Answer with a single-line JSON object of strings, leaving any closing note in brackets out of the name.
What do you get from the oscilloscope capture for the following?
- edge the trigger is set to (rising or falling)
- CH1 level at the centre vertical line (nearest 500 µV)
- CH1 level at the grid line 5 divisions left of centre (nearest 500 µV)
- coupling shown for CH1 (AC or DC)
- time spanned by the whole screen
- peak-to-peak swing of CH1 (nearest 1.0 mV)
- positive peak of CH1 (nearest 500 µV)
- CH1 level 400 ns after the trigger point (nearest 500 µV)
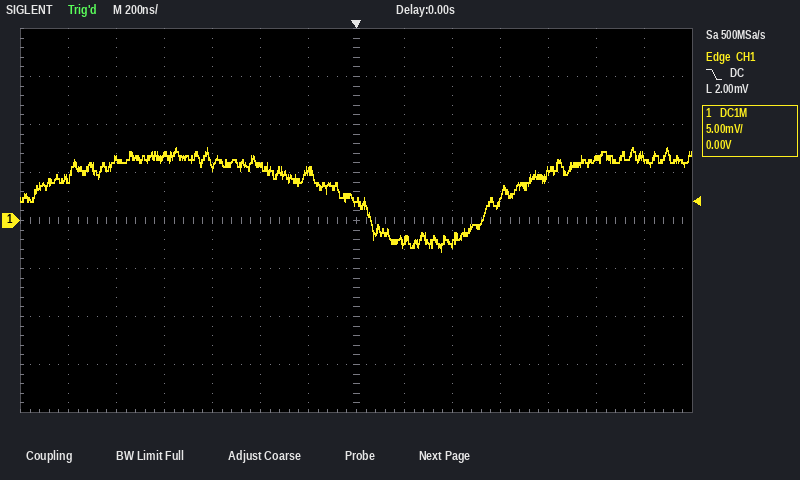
{"edge the trigger is set to": "falling", "CH1 level at the centre vertical line": "2.0 mV", "CH1 level at the grid line 5 divisions left of centre": "6.5 mV", "coupling shown for CH1": "DC", "time spanned by the whole screen": "2.8 µs", "peak-to-peak swing of CH1": "11.0 mV", "positive peak of CH1": "7.5 mV", "CH1 level 400 ns after the trigger point": "-2.5 mV"}
